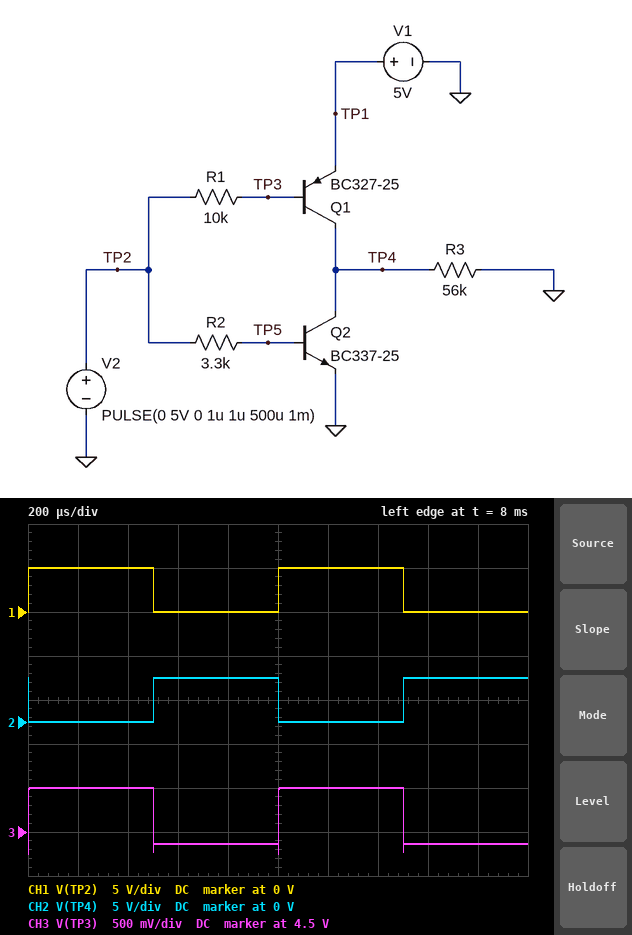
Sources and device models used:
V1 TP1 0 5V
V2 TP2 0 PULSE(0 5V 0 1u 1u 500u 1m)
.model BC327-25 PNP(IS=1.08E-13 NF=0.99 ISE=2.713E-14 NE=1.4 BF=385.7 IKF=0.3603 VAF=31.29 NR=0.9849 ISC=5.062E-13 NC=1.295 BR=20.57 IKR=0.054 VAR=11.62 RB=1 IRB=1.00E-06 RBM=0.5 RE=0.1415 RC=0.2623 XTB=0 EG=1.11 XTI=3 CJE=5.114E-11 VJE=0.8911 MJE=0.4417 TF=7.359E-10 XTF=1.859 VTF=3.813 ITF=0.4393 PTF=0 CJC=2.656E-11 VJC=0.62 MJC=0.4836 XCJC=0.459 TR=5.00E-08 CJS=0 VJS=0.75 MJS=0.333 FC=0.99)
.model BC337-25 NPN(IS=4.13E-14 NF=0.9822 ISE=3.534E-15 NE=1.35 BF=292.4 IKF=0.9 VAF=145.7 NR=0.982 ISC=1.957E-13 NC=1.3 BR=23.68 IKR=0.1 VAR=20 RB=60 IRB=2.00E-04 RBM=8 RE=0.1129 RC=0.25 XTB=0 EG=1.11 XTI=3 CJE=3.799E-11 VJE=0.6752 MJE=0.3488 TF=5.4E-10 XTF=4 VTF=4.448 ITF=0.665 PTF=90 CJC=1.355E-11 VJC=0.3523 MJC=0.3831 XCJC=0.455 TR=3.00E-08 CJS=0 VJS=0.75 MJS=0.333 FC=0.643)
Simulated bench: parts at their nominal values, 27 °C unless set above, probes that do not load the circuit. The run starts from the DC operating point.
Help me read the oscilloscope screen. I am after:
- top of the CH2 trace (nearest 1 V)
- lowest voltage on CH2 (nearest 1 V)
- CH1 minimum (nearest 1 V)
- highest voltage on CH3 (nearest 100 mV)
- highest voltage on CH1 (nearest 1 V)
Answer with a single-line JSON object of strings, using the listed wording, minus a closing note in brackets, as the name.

{"top of the CH2 trace": "5 V", "lowest voltage on CH2": "0 V", "CH1 minimum": "0 V", "highest voltage on CH3": "5.0 V", "highest voltage on CH1": "5 V"}
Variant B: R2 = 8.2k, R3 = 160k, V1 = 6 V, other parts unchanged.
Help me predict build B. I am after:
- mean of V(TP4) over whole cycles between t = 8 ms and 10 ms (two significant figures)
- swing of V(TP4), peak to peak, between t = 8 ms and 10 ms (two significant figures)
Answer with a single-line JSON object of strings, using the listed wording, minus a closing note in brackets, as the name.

{"mean of V(TP4) over whole cycles between t = 8 ms and 10 ms": "3.0 V", "swing of V(TP4), peak to peak, between t = 8 ms and 10 ms": "6.0 V"}
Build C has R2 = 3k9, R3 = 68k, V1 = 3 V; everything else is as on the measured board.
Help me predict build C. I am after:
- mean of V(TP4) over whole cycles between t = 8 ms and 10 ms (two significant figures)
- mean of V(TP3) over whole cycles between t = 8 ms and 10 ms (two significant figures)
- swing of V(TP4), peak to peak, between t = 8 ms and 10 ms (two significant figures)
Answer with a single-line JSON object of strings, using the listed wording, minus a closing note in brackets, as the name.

{"mean of V(TP4) over whole cycles between t = 8 ms and 10 ms": "1.5 V", "mean of V(TP3) over whole cycles between t = 8 ms and 10 ms": "3.7 V", "swing of V(TP4), peak to peak, between t = 8 ms and 10 ms": "3.0 V"}
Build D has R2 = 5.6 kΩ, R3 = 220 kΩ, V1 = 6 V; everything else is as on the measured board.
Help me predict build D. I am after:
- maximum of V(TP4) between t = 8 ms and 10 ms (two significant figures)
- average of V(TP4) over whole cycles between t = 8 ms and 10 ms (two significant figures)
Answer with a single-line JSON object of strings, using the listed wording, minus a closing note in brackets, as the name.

{"maximum of V(TP4) between t = 8 ms and 10 ms": "6.0 V", "average of V(TP4) over whole cycles between t = 8 ms and 10 ms": "3.0 V"}
